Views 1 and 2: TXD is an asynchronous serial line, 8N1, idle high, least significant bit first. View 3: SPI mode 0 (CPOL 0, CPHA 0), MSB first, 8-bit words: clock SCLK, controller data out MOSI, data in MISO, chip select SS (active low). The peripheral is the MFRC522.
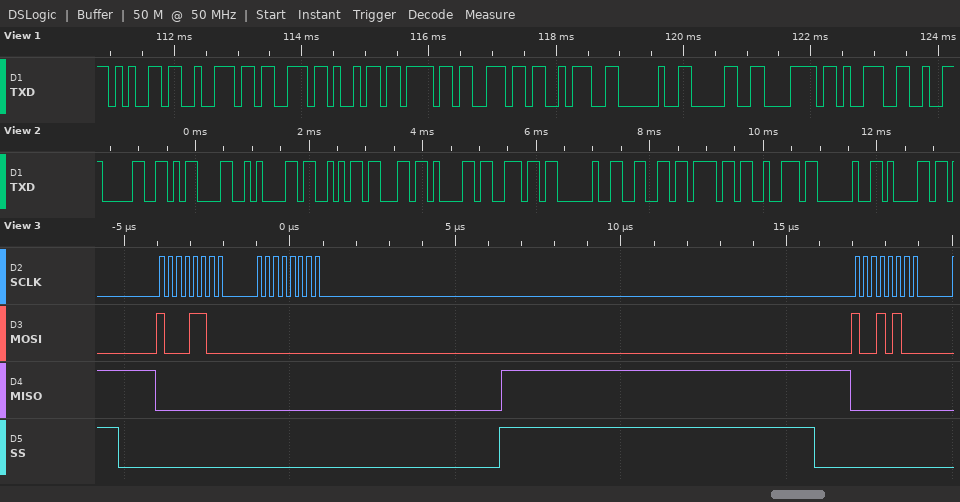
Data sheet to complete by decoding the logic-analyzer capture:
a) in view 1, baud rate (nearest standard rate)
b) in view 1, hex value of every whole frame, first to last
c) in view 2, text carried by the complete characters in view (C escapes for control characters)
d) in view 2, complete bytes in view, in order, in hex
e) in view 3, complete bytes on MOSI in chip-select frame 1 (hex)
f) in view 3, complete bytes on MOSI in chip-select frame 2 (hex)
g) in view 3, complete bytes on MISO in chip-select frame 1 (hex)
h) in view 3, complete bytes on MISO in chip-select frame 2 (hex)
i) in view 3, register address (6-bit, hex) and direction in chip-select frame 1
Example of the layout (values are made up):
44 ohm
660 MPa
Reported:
9600 baud
65 72 73 69 6F 6E 3A 20 30 78 39
"0\r\nScan for a"
30 0D 0A 53 63 61 6E 20 66 6F 72 20 61
8C 00
94
00 00
00
0x06 read
